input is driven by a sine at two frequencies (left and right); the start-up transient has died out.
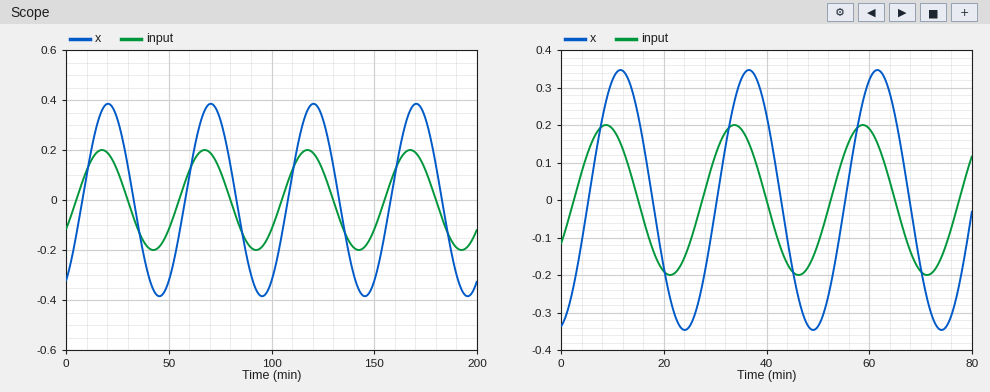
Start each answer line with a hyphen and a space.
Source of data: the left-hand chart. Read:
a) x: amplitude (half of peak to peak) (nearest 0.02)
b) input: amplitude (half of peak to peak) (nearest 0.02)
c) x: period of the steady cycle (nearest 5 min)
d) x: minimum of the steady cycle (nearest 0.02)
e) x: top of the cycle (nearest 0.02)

- 0.38
- 0.20
- 50 min
- -0.38
- 0.38
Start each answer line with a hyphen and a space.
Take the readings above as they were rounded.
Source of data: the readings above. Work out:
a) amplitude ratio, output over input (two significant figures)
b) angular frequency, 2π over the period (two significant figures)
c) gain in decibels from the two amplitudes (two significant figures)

- 1.9
- 0.13 rad/min
- 5.6 dB
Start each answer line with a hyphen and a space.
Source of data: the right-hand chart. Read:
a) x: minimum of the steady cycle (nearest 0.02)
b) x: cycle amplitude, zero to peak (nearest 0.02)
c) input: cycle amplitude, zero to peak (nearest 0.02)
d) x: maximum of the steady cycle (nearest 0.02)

- -0.34
- 0.34
- 0.20
- 0.34
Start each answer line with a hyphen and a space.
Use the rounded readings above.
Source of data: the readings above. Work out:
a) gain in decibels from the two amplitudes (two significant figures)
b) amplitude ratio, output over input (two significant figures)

- 4.6 dB
- 1.7
